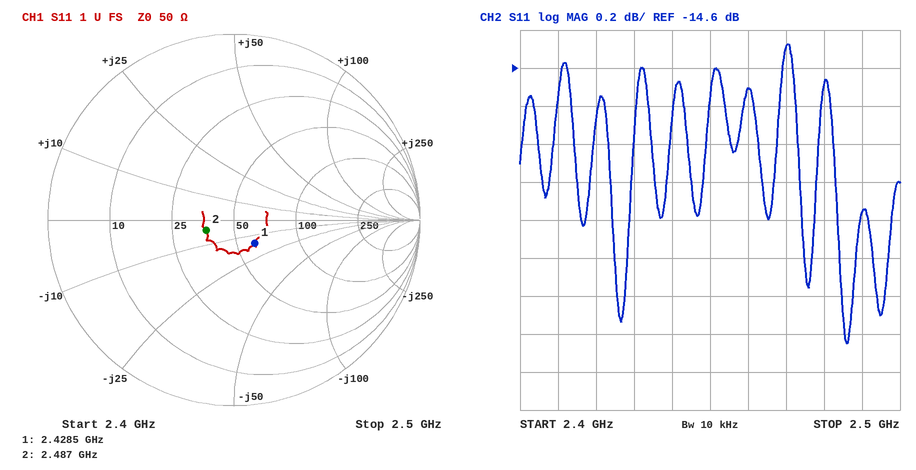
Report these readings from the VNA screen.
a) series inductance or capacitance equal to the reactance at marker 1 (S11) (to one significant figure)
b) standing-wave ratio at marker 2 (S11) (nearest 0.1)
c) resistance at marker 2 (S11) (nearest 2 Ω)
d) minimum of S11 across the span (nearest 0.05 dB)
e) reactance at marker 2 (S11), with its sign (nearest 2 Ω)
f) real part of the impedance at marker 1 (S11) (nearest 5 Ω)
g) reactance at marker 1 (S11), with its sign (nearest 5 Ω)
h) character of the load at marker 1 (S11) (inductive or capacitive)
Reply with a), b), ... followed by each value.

a) 4 pF
b) 1.4
c) 36 Ω
d) -16.05 dB
e) -4 Ω
f) 60 Ω
g) -15 Ω
h) capacitive
